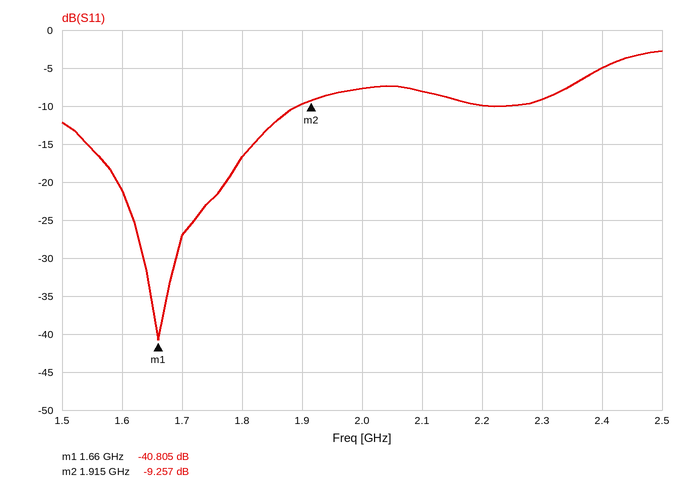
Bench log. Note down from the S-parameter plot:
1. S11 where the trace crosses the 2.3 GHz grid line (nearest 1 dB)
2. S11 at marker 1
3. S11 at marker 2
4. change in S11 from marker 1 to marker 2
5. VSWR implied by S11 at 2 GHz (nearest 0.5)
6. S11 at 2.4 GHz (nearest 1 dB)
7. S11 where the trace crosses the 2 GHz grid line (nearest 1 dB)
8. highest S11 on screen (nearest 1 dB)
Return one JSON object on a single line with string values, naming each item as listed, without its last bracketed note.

{"S11 where the trace crosses the 2.3 GHz grid line": "-9 dB", "S11 at marker 1": "-40.805 dB", "S11 at marker 2": "-9.257 dB", "change in S11 from marker 1 to marker 2": "31.548 dB", "VSWR implied by S11 at 2 GHz": "2.5", "S11 at 2.4 GHz": "-5 dB", "S11 where the trace crosses the 2 GHz grid line": "-8 dB", "highest S11 on screen": "-3 dB"}
